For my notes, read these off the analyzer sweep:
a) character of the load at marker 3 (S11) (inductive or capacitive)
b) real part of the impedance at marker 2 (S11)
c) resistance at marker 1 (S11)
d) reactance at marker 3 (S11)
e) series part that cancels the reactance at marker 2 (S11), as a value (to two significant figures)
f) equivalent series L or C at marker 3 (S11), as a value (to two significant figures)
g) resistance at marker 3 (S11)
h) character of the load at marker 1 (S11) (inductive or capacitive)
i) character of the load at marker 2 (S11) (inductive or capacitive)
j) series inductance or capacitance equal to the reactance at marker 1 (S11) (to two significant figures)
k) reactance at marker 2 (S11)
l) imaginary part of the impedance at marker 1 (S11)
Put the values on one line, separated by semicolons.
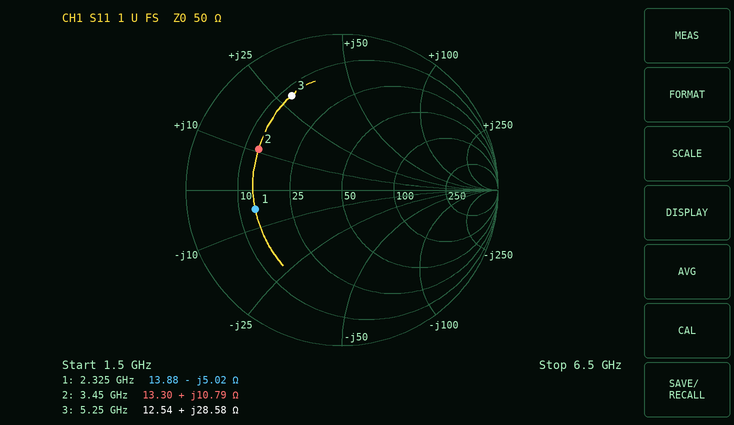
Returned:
inductive; 13.30 Ω; 13.88 Ω; +28.58 Ω; 4.3 pF; 870 pH; 12.54 Ω; capacitive; inductive; 14 pF; +10.79 Ω; -5.02 Ω
